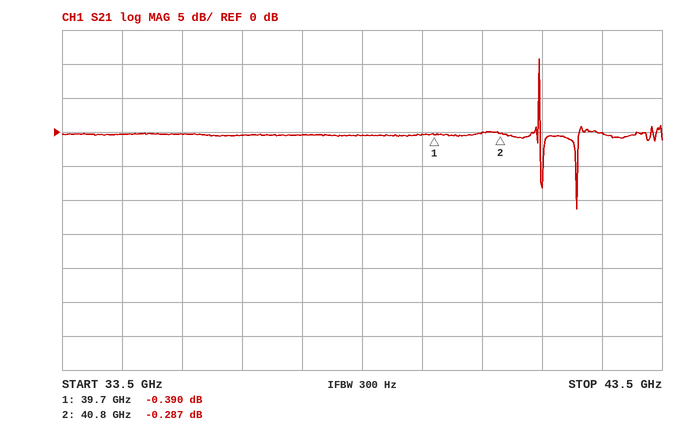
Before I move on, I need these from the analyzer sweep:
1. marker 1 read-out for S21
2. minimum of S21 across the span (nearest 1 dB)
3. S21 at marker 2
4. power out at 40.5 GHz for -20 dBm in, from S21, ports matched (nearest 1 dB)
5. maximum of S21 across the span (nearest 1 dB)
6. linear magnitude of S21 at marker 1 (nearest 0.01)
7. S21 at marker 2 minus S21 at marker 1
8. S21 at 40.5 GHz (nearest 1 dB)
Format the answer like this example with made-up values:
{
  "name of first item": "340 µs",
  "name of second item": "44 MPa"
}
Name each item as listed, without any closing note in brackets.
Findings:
{
  "marker 1 read-out for S21": "-0.390 dB",
  "minimum of S21 across the span": "-11 dB",
  "S21 at marker 2": "-0.287 dB",
  "power out at 40.5 GHz for -20 dBm in, from S21, ports matched": "-20 dBm",
  "maximum of S21 across the span": "11 dB",
  "linear magnitude of S21 at marker 1": "0.96",
  "S21 at marker 2 minus S21 at marker 1": "0.103 dB",
  "S21 at 40.5 GHz": "0 dB"
}
